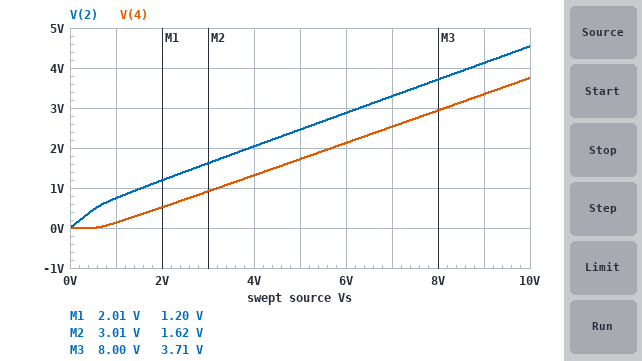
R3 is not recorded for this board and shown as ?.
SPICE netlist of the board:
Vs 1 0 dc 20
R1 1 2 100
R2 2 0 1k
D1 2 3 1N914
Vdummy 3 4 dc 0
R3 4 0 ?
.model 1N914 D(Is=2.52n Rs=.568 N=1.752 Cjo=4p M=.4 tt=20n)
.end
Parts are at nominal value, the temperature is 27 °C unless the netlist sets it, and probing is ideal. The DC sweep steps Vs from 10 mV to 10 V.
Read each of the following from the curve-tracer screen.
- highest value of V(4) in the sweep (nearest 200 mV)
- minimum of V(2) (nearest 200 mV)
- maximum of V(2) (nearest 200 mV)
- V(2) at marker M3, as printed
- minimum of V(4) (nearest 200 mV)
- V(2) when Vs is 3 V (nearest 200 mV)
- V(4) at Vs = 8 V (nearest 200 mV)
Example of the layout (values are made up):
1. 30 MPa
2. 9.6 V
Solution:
1. 3.8 V
2. 0 V
3. 4.6 V
4. 3.71 V
5. 0 V
6. 1.6 V
7. 3.0 V
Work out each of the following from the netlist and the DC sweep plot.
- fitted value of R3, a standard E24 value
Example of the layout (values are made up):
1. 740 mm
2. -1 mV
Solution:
1. 75 Ω
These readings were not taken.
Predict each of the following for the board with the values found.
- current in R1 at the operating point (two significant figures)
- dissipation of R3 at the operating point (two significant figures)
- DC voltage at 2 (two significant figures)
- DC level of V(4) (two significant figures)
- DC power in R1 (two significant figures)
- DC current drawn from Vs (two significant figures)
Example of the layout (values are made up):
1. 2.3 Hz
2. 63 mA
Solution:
1. 110 mA
2. 820 mW
3. 8.7 V
4. 7.8 V
5. 1.3 W
6. 110 mA
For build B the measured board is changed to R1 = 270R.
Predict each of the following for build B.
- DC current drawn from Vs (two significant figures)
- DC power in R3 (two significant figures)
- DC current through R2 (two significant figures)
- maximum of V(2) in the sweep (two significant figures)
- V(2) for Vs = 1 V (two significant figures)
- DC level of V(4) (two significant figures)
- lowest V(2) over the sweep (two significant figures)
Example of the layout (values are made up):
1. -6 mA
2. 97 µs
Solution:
1. 57 mA
2. 200 mW
3. 4.7 mA
4. 2.6 V
5. 630 mV
6. 3.9 V
7. 7.9 mV
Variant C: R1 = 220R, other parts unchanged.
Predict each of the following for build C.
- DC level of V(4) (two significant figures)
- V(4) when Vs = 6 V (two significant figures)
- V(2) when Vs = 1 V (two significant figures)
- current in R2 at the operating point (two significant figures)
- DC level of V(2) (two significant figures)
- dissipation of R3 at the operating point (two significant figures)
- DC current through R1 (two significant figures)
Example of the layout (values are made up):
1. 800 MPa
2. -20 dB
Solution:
1. 4.6 V
2. 1.2 V
3. 650 mV
4. 5.4 mA
5. 5.4 V
6. 280 mW
7. 66 mA
